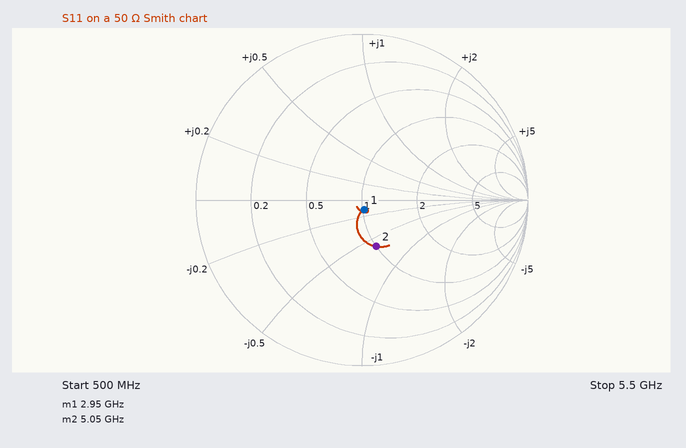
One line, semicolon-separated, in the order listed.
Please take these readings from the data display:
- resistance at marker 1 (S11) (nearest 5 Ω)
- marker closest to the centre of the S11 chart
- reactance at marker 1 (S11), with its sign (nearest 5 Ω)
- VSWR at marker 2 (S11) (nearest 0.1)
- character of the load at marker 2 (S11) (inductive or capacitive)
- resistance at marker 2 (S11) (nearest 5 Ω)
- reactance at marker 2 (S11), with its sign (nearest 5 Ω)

50 Ω; marker 1; -5 Ω; 1.8; capacitive; 50 Ω; -30 Ω
